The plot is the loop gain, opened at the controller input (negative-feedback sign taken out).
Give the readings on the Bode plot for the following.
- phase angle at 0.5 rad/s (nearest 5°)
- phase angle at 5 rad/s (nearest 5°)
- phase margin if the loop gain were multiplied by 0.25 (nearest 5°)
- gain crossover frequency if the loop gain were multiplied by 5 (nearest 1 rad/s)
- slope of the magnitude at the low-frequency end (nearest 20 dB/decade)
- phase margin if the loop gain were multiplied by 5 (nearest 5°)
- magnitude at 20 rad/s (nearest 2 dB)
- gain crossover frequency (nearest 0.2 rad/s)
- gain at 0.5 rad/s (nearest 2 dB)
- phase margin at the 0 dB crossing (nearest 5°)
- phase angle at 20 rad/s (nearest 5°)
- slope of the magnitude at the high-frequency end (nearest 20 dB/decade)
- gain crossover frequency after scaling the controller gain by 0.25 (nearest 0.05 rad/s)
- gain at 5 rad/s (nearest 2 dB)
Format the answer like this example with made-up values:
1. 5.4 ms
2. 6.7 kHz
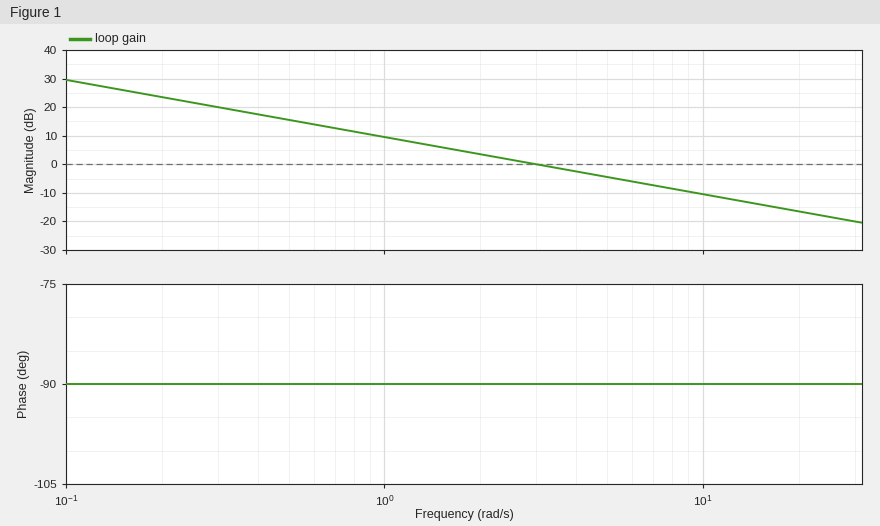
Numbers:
1. -90°
2. -90°
3. 90°
4. 15 rad/s
5. -20 dB/decade
6. 90°
7. -16 dB
8. 3.0 rad/s
9. 16 dB
10. 90°
11. -90°
12. -20 dB/decade
13. 0.75 rad/s
14. -4 dB
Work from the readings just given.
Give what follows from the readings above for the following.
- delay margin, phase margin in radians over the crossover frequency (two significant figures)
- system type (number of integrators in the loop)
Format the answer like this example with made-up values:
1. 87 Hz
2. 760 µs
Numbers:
1. 0.52 s
2. 1
